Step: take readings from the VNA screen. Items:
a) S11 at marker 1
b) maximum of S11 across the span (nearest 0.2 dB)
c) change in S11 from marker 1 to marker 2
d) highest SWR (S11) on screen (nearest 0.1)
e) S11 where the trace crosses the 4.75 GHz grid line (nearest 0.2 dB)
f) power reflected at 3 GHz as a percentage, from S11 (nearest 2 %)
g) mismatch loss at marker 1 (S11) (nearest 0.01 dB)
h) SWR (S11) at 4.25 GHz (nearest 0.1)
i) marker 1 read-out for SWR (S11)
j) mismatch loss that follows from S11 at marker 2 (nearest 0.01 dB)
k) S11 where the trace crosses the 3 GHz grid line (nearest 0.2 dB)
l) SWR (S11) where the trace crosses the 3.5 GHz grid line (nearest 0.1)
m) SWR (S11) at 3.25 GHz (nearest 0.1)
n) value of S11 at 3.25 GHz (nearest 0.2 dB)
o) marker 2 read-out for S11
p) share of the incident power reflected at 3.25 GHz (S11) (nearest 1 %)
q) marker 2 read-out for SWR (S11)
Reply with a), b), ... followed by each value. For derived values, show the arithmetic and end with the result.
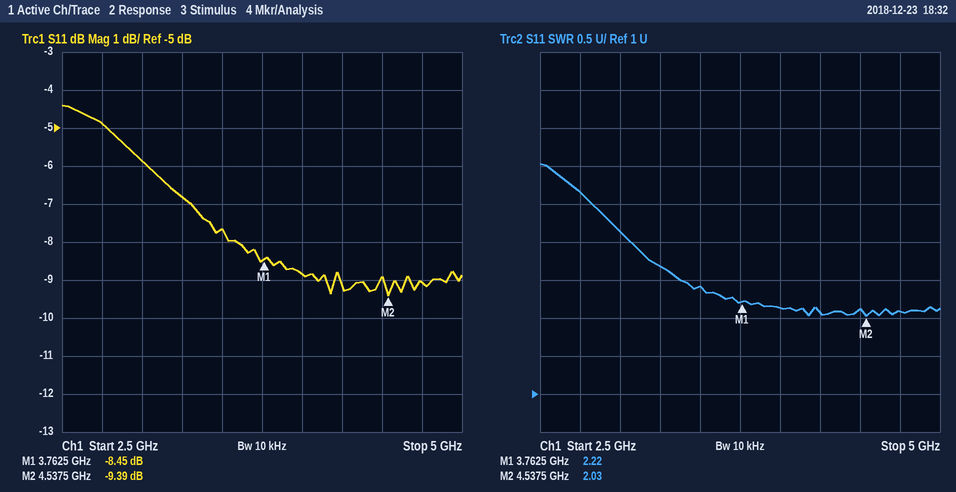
a) -8.45 dB
b) -4.4 dB
c) -9.39 − (-8.45) = -0.94 dB
d) 4.0
e) -9.0 dB
f) 10^(-5.8/10) ≈ 26 %
g) −10 log10(1 − 10^(-8.45/10)) ≈ 0.67 dB
h) 2.1
i) 2.22
j) −10 log10(1 − 10^(-9.39/10)) ≈ 0.53 dB
k) -5.8 dB
l) 2.4
m) 2.7
n) -6.8 dB
o) -9.39 dB
p) 10^(-6.8/10) ≈ 21 %
q) 2.03
